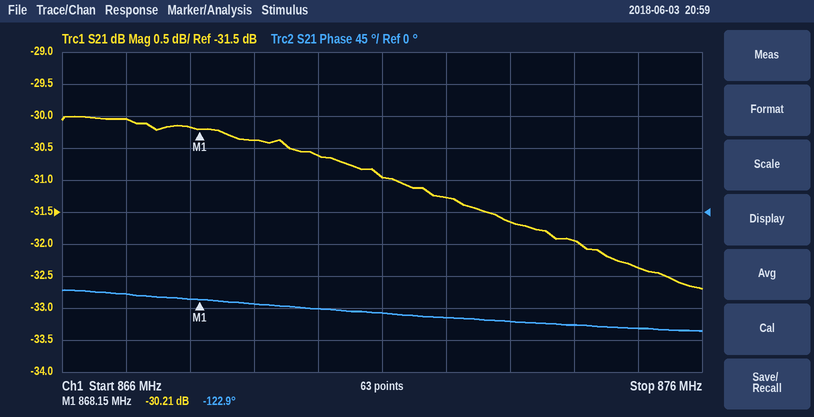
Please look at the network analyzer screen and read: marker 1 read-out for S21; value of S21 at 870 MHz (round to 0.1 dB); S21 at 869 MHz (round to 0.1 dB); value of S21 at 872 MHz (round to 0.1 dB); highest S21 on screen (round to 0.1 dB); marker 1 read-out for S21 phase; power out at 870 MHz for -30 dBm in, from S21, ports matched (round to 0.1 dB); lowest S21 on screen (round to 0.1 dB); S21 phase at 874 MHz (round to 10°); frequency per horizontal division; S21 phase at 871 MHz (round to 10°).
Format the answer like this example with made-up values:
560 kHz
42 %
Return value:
-30.21 dB
-30.6 dB
-30.4 dB
-31.3 dB
-30.0 dB
-122.9°
-60.6 dBm
-32.7 dB
-160°
1 MHz
-140°
